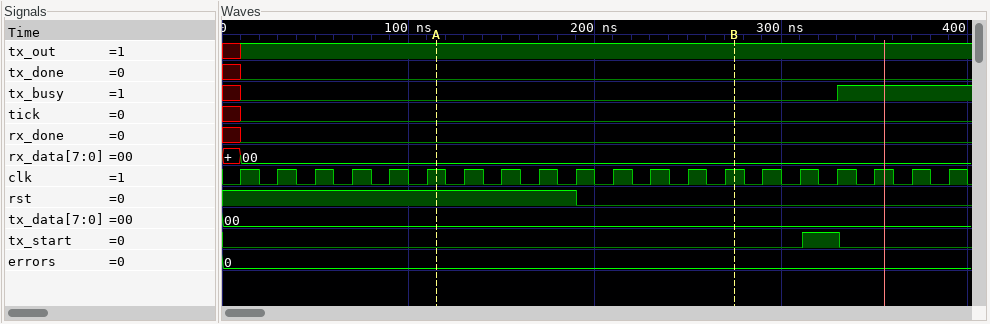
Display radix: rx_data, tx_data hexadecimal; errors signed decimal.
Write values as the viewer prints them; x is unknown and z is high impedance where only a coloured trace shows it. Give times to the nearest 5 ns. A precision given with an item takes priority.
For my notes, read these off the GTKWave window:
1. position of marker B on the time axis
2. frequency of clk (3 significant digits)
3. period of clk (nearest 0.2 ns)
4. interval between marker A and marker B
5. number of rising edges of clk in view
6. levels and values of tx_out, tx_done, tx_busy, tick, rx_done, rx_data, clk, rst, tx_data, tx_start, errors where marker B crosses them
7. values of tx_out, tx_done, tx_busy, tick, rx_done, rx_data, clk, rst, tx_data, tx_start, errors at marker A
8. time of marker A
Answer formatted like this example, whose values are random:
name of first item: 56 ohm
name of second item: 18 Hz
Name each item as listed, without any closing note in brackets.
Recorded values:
position of marker B on the time axis: 275 ns
frequency of clk: 50.0 MHz
period of clk: 20 ns
interval between marker A and marker B: 160 ns
number of rising edges of clk in view: 20
levels and values of tx_out, tx_done, tx_busy, tick, rx_done, rx_data, clk, rst, tx_data, tx_start, errors where marker B crosses them: tx_out=1, tx_done=0, tx_busy=0, tick=0, rx_done=0, rx_data=00, clk=1, rst=0, tx_data=00, tx_start=0, errors=0
values of tx_out, tx_done, tx_busy, tick, rx_done, rx_data, clk, rst, tx_data, tx_start, errors at marker A: tx_out=1, tx_done=0, tx_busy=0, tick=0, rx_done=0, rx_data=00, clk=1, rst=1, tx_data=00, tx_start=0, errors=0
time of marker A: 115 ns
